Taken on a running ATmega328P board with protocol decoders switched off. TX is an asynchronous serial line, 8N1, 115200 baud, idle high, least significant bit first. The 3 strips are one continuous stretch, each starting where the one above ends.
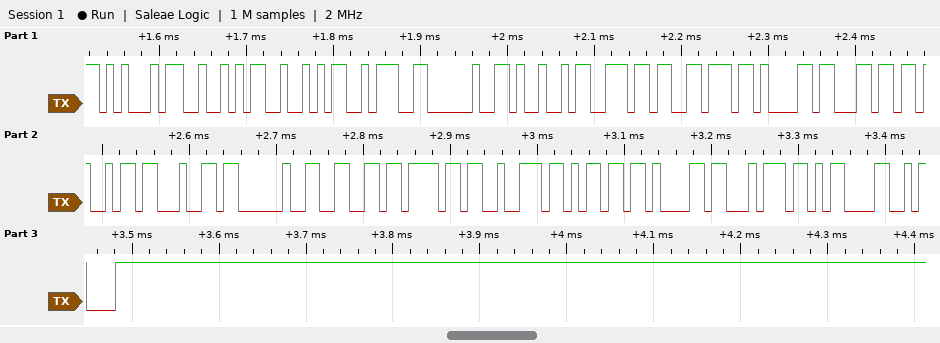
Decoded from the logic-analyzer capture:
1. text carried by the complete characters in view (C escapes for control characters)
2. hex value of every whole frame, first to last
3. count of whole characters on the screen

"ERR: Invalid format\r\n"
45 52 52 3A 20 49 6E 76 61 6C 69 64 20 66 6F 72 6D 61 74 0D 0A
21
